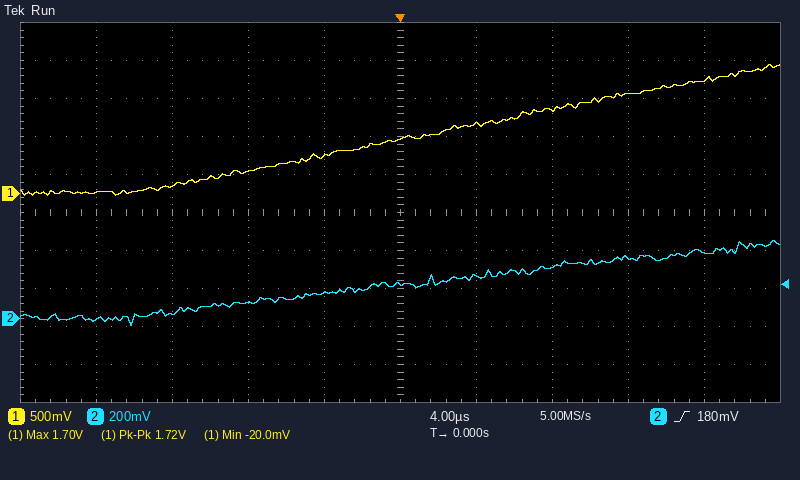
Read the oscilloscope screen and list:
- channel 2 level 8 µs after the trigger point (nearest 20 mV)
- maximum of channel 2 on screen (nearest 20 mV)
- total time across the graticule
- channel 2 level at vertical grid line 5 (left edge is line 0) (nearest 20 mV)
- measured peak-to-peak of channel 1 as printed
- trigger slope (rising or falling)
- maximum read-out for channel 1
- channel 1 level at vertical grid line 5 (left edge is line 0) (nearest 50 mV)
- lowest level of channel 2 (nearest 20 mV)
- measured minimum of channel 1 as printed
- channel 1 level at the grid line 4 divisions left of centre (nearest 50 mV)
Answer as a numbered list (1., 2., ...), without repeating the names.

1. 280 mV
2. 420 mV
3. 40 µs
4. 180 mV
5. 1.72 V
6. rising
7. 1.70 V
8. 700 mV
9. -40 mV
10. -20.0 mV
11. 0 mV
